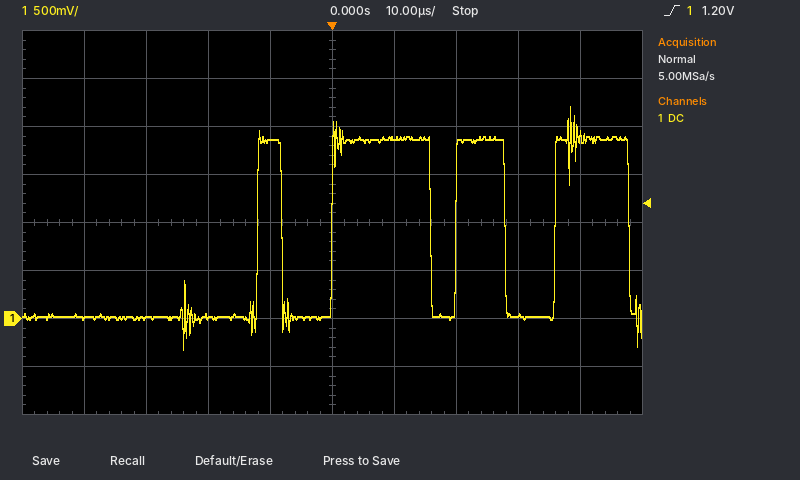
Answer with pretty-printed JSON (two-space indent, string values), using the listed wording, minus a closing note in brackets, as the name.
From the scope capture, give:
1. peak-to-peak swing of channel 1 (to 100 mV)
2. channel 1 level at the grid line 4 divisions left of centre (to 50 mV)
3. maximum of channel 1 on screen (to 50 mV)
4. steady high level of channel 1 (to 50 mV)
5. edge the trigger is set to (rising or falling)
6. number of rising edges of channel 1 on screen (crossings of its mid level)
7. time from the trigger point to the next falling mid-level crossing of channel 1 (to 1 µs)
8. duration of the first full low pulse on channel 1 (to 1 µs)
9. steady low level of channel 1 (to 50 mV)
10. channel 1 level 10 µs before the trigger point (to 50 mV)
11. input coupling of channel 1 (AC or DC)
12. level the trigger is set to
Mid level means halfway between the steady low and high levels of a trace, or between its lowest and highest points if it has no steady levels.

{
  "peak-to-peak swing of channel 1": "2.50 V",
  "channel 1 level at the grid line 4 divisions left of centre": "0 mV",
  "maximum of channel 1 on screen": "2.20 V",
  "steady high level of channel 1": "1.85 V",
  "edge the trigger is set to": "rising",
  "number of rising edges of channel 1 on screen": "4",
  "time from the trigger point to the next falling mid-level crossing of channel 1": "16 µs",
  "duration of the first full low pulse on channel 1": "8 µs",
  "steady low level of channel 1": "0 mV",
  "channel 1 level 10 µs before the trigger point": "1.85 V",
  "input coupling of channel 1": "DC",
  "level the trigger is set to": "1.20 V"
}
